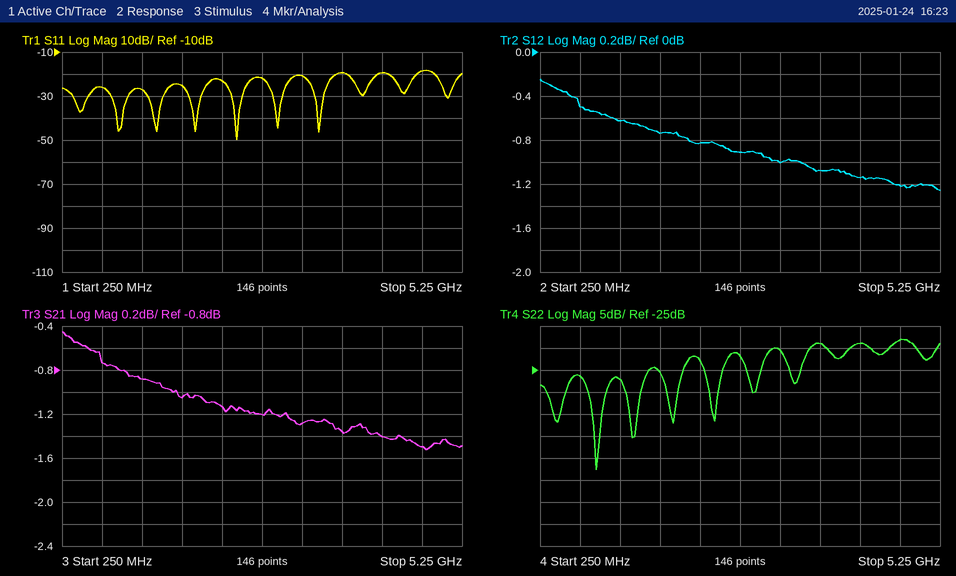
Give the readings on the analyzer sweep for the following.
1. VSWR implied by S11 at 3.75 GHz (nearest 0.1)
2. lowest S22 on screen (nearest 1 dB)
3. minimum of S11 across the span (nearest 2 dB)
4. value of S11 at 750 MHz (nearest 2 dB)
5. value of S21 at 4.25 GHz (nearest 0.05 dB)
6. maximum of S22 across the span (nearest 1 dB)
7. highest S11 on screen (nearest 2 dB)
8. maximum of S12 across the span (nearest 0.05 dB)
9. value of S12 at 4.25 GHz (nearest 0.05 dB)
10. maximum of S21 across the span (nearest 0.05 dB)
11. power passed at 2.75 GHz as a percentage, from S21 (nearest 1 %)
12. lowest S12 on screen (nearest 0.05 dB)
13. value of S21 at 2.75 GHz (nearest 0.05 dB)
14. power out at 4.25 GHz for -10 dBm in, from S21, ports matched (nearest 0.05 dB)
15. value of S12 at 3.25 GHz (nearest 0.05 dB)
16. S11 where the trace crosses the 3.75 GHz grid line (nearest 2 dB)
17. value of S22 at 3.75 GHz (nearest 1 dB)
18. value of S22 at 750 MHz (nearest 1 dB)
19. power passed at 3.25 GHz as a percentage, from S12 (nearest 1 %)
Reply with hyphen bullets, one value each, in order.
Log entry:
- 1.2
- -48 dB
- -50 dB
- -26 dB
- -1.40 dB
- -18 dB
- -18 dB
- -0.25 dB
- -1.15 dB
- -0.45 dB
- 76 %
- -1.25 dB
- -1.20 dB
- -11.40 dBm
- -1.00 dB
- -20 dB
- -19 dB
- -26 dB
- 79 %
